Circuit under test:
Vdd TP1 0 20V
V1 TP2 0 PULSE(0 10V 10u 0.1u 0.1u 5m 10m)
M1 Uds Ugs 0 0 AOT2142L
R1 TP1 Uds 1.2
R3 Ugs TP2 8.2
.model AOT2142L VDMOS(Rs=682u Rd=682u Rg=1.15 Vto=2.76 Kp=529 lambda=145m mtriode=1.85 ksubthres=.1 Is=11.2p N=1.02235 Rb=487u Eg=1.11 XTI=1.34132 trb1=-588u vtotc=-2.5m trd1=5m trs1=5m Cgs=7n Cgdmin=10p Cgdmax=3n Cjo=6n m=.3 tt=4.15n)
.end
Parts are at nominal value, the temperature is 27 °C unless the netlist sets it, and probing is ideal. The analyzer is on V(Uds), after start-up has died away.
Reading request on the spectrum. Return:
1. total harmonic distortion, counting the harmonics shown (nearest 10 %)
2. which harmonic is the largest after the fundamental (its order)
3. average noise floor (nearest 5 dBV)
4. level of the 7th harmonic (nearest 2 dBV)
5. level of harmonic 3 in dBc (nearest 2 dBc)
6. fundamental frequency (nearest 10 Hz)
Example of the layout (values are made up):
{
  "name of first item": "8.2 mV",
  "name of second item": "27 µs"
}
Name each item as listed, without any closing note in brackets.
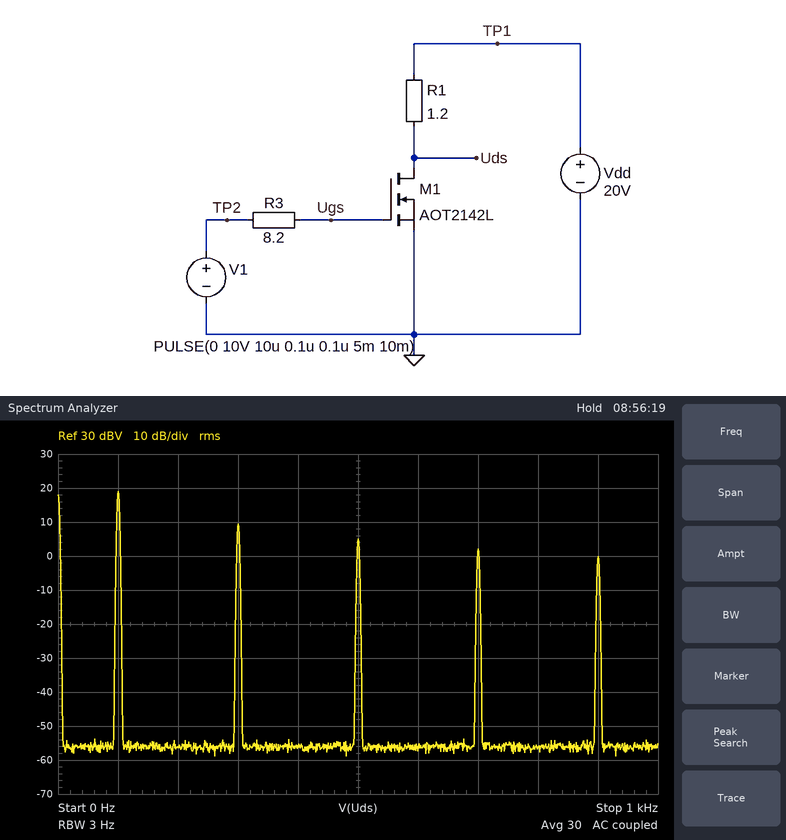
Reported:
{
  "total harmonic distortion, counting the harmonics shown": "40 %",
  "which harmonic is the largest after the fundamental": "3",
  "average noise floor": "-55 dBV",
  "level of the 7th harmonic": "2 dBV",
  "level of harmonic 3 in dBc": "-10 dBc",
  "fundamental frequency": "100 Hz"
}
